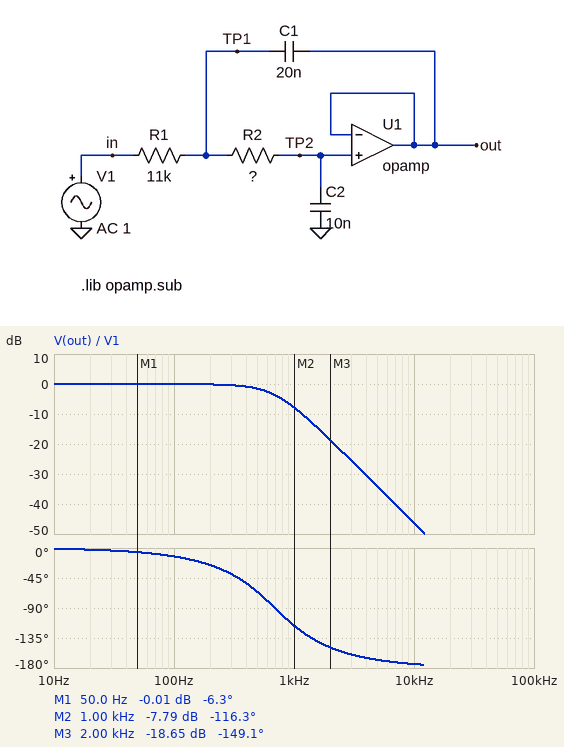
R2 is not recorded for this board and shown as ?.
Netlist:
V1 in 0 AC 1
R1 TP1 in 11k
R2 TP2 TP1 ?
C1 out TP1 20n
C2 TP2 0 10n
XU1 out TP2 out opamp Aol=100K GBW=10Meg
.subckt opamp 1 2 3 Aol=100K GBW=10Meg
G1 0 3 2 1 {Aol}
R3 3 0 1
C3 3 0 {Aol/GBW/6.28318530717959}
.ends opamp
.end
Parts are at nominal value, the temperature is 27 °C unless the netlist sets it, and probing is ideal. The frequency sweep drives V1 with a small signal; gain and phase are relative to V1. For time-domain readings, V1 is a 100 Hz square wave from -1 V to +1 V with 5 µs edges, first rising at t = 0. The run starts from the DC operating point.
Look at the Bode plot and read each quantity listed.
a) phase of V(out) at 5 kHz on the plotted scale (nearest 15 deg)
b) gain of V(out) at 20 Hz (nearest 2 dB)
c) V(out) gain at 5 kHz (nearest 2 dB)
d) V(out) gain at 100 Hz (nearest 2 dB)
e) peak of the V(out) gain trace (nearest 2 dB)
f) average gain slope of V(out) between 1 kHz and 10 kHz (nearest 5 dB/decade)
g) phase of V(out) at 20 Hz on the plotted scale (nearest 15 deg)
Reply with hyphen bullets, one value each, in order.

- -165 deg
- 0 dB
- -34 dB
- 0 dB
- 0 dB
- -40 dB/decade
- 0 deg
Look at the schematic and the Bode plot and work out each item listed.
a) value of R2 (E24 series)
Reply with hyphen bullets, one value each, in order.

- 24 kΩ
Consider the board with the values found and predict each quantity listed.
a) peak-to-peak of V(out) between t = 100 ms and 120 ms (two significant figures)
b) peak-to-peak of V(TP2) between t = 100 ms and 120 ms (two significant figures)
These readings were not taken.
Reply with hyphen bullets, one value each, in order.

- 2.1 V
- 2.1 V
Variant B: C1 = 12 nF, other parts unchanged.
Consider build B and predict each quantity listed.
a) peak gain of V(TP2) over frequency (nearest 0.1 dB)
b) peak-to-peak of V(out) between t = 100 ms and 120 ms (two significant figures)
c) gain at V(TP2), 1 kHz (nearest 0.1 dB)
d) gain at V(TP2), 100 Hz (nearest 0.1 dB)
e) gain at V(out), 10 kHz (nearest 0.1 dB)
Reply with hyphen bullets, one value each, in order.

- 0 dB
- 2.0 V
- -6.9 dB
- -0.1 dB
- -42.0 dB
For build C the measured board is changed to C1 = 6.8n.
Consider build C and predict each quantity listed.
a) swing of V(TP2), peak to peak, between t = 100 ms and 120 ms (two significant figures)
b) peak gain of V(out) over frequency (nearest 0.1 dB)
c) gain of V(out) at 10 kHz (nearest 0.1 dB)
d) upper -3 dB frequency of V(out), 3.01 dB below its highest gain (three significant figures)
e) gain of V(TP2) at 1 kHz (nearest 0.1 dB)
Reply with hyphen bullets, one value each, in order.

- 2.0 V
- 0 dB
- -37.3 dB
- 530 Hz
- -6.9 dB
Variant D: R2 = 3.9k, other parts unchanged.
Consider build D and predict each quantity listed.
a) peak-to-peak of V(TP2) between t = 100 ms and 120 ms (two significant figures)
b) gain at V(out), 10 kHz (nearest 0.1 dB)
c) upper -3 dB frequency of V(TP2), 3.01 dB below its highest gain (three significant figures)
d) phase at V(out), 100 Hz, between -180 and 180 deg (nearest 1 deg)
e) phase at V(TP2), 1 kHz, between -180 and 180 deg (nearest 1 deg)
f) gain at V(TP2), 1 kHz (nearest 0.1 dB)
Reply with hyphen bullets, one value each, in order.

- 2.1 V
- -30.7 dB
- 1.49 kHz
- -5 deg
- -55 deg
- -1.2 dB
